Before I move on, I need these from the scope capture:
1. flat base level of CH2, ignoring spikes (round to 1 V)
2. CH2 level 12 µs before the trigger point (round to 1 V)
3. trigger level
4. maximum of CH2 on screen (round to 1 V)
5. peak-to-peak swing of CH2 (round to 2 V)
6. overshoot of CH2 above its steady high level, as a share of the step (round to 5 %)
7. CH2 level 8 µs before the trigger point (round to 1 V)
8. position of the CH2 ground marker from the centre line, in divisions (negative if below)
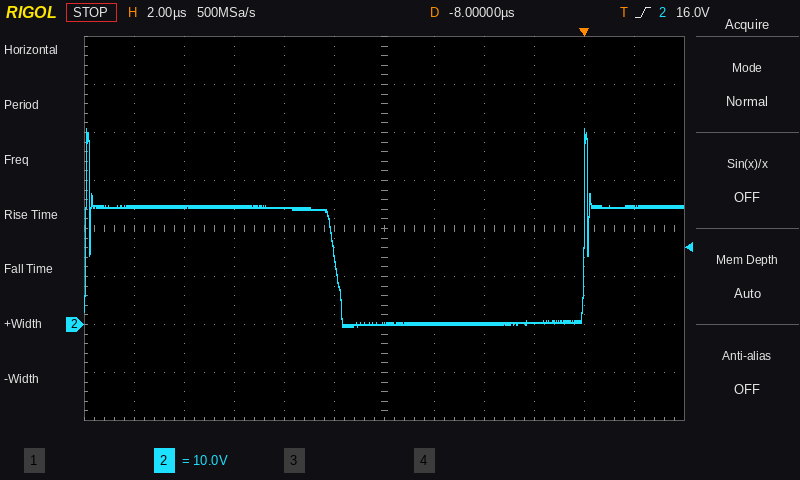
0 V
24 V
16.0 V
41 V
42 V
65 %
0 V
-2.0 div
